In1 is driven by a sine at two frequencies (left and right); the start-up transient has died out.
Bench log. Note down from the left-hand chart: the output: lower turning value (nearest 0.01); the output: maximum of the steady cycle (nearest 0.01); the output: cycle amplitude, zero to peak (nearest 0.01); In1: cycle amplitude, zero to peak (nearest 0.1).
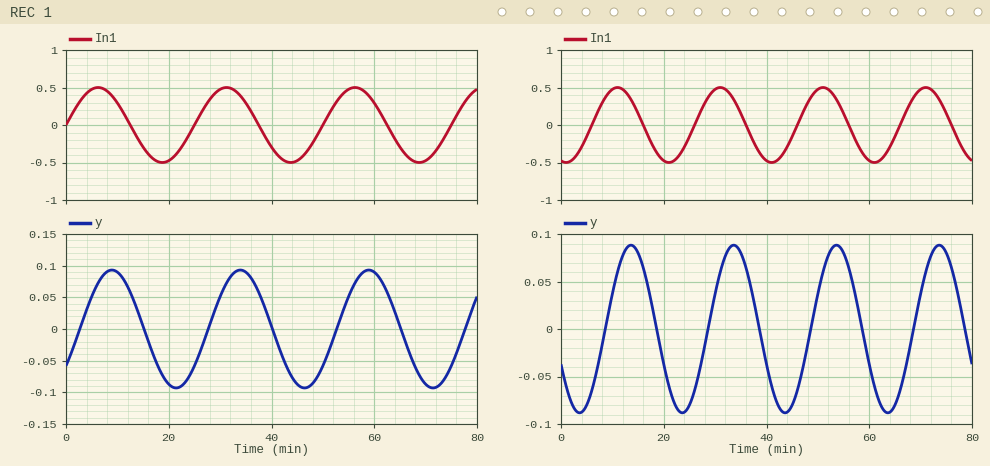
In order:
-0.09
0.09
0.09
0.5
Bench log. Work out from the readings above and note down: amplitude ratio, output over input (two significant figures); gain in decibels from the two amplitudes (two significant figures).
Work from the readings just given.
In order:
0.18
-15 dB
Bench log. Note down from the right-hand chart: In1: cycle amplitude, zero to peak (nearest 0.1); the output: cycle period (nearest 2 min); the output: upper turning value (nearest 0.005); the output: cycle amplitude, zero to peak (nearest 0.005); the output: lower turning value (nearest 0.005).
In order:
0.5
20 min
0.090
0.090
-0.090
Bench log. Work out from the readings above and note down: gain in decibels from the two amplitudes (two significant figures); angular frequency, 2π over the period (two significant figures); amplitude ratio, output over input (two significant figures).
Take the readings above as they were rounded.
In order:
-15 dB
0.31 rad/min
0.18
